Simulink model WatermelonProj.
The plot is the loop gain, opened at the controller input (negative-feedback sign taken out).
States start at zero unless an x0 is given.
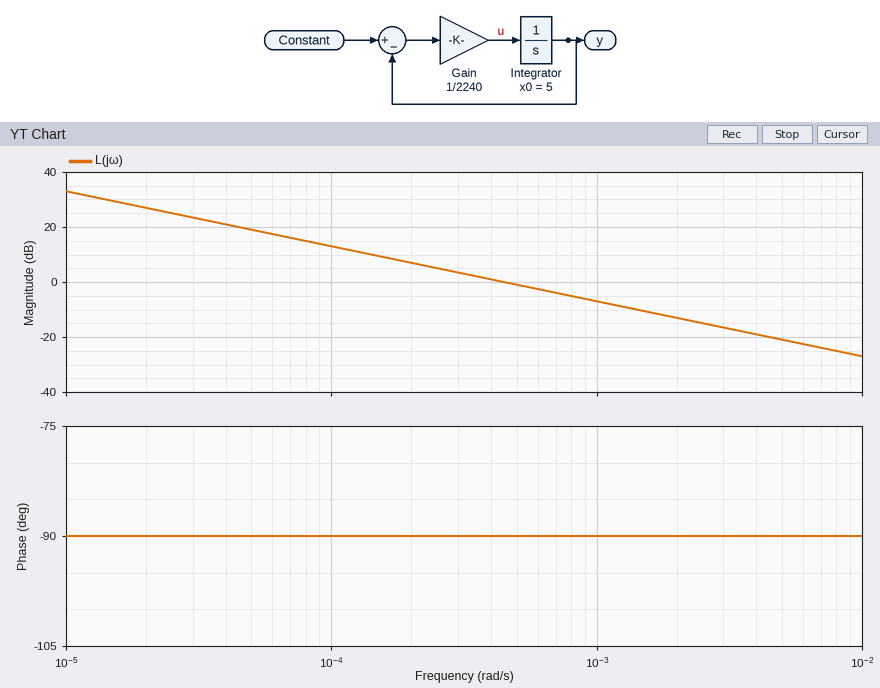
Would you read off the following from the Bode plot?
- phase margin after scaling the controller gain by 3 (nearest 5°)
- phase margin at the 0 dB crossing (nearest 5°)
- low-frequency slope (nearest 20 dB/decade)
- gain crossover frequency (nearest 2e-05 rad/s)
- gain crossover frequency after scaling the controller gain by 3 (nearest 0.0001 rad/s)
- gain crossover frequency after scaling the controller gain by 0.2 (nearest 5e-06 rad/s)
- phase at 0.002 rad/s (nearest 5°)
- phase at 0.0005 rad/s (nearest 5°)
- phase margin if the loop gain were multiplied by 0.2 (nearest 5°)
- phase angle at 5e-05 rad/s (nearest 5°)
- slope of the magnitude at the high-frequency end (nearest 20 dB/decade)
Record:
90°
90°
-20 dB/decade
0.00044 rad/s
0.0013 rad/s
0.000090 rad/s
-90°
-90°
90°
-90°
-20 dB/decade
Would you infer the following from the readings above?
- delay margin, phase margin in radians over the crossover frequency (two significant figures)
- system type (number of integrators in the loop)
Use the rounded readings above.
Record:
3600 s
1
